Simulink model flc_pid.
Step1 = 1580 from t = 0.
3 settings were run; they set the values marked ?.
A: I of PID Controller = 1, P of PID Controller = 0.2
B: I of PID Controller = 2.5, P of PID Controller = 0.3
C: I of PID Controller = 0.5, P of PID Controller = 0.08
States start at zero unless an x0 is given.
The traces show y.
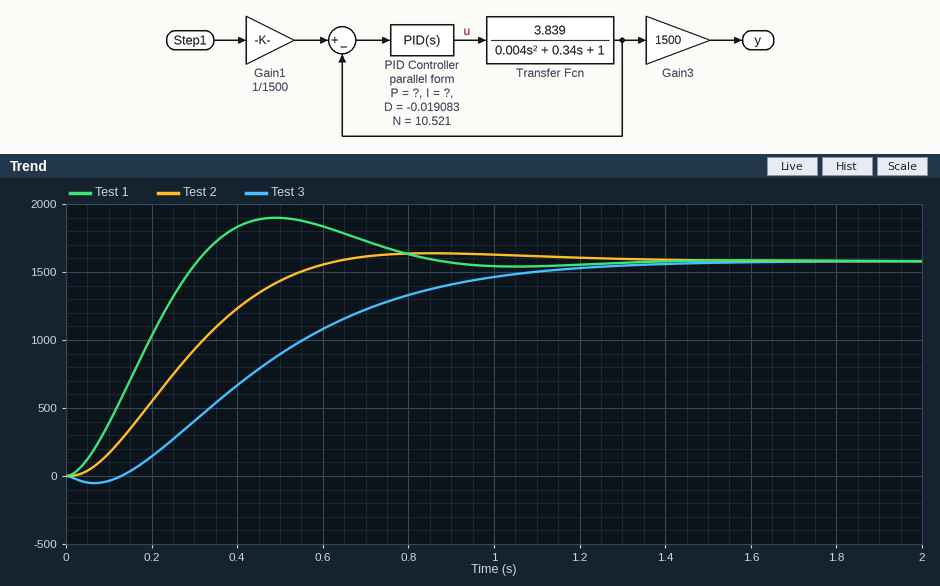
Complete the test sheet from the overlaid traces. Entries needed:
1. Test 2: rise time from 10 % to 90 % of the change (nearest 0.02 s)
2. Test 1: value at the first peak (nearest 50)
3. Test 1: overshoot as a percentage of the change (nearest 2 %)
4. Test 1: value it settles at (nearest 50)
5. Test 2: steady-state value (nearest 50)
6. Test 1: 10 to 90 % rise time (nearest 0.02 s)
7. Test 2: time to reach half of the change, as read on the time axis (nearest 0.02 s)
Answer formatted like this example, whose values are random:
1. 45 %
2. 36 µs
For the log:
1. 0.40 s
2. 1900
3. 20 %
4. 1600
5. 1600
6. 0.22 s
7. 0.26 s
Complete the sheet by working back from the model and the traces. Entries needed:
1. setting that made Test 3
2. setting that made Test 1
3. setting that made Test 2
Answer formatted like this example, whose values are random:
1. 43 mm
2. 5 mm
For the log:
1. C
2. B
3. A
